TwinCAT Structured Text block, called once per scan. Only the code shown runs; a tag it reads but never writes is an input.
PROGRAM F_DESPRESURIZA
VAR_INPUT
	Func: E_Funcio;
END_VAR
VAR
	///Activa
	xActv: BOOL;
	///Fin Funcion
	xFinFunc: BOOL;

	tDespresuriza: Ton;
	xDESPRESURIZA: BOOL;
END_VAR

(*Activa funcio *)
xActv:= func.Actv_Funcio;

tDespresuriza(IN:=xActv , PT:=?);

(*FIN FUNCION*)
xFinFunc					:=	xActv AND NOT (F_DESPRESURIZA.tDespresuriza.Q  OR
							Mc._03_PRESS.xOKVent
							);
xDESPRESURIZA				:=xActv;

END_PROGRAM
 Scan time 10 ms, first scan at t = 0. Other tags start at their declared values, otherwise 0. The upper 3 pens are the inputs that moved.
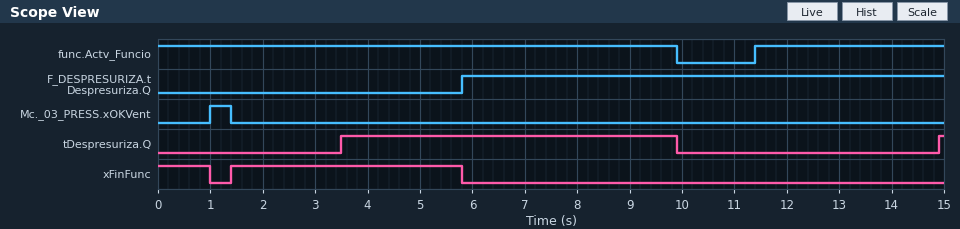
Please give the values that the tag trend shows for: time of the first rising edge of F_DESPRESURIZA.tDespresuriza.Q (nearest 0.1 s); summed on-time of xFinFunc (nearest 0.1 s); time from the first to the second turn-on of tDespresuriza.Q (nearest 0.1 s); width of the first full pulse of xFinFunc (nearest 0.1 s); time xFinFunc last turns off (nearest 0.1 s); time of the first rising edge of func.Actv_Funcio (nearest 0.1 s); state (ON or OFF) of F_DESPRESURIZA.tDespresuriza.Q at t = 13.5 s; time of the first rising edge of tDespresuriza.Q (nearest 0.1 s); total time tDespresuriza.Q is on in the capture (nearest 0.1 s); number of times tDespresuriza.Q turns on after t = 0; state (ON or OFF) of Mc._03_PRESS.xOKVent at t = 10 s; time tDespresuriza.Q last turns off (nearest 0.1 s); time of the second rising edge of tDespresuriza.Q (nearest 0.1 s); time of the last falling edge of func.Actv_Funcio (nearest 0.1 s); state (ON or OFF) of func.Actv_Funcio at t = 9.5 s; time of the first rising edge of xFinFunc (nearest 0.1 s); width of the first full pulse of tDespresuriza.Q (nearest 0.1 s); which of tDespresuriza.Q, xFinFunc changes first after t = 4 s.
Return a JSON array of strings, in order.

["5.8 s", "5.4 s", "11.4 s", "4.4 s", "5.8 s", "11.4 s", "ON", "3.5 s", "6.5 s", "2", "OFF", "9.9 s", "14.9 s", "9.9 s", "ON", "1.4 s", "6.4 s", "xFinFunc"]
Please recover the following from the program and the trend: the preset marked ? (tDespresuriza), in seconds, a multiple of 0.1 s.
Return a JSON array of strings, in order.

["3.5 s"]
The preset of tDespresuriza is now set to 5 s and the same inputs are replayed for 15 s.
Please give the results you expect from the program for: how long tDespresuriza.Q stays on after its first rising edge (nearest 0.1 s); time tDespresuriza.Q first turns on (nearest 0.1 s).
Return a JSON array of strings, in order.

["4.9 s", "5.0 s"]
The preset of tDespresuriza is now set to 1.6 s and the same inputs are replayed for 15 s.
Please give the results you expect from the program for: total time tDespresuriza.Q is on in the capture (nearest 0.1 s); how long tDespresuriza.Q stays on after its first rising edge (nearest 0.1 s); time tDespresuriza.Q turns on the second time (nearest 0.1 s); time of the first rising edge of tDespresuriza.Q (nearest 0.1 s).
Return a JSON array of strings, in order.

["10.3 s", "8.3 s", "13.0 s", "1.6 s"]
